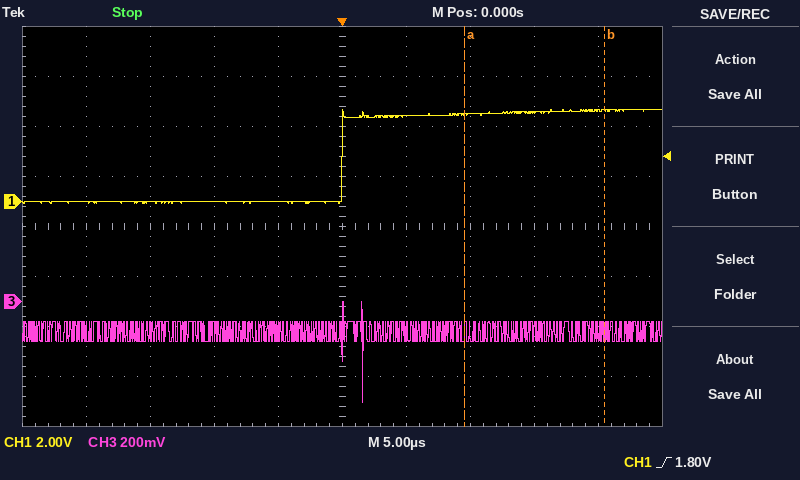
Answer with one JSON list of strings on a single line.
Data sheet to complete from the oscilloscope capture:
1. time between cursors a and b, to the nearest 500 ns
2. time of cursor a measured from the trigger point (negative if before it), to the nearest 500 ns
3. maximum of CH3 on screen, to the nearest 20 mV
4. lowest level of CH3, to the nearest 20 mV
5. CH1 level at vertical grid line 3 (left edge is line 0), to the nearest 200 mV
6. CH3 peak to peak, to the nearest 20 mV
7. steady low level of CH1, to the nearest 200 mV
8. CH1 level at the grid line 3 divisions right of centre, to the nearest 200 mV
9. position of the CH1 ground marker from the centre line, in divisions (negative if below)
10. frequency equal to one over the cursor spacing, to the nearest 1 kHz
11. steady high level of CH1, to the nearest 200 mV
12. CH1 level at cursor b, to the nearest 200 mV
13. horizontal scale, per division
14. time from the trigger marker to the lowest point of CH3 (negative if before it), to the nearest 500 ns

["11.0 µs", "+9.5 µs", "0 mV", "-400 mV", "0.0 V", "400 mV", "0.0 V", "3.6 V", "+0.5 div", "91 kHz", "3.6 V", "3.6 V", "5 µs", "+1.5 µs"]
